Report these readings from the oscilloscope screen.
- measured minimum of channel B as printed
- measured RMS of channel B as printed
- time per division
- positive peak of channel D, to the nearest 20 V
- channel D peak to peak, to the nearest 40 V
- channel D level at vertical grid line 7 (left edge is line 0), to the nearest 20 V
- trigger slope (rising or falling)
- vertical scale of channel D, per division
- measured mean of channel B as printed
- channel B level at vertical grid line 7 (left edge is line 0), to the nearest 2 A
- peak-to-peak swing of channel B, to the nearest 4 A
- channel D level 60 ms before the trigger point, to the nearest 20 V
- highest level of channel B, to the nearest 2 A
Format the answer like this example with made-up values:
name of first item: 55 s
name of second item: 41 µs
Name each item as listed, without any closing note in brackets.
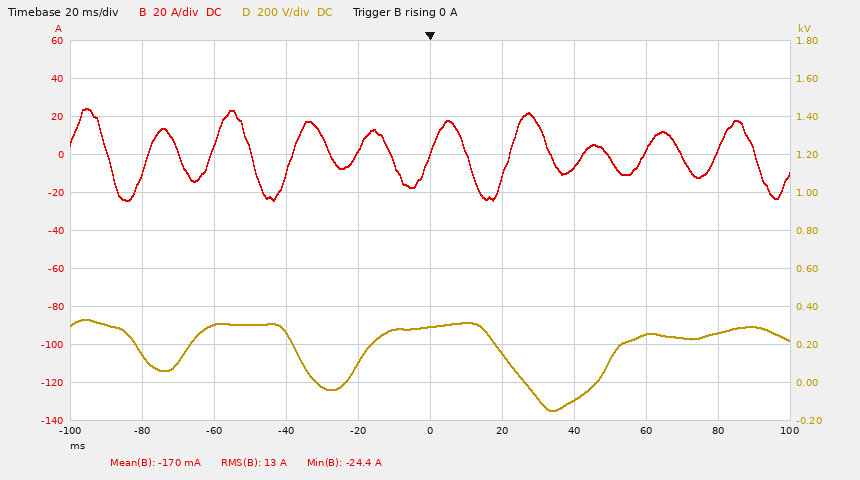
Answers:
measured minimum of channel B as printed: -24.4 A
measured RMS of channel B as printed: 13 A
time per division: 20 ms
positive peak of channel D, to the nearest 20 V: 340 V
channel D peak to peak, to the nearest 40 V: 480 V
channel D level at vertical grid line 7 (left edge is line 0), to the nearest 20 V: -100 V
trigger slope: rising
vertical scale of channel D, per division: 200 V
measured mean of channel B as printed: -170 mA
channel B level at vertical grid line 7 (left edge is line 0), to the nearest 2 A: -6 A
peak-to-peak swing of channel B, to the nearest 4 A: 48 A
channel D level 60 ms before the trigger point, to the nearest 20 V: 300 V
highest level of channel B, to the nearest 2 A: 24 A
